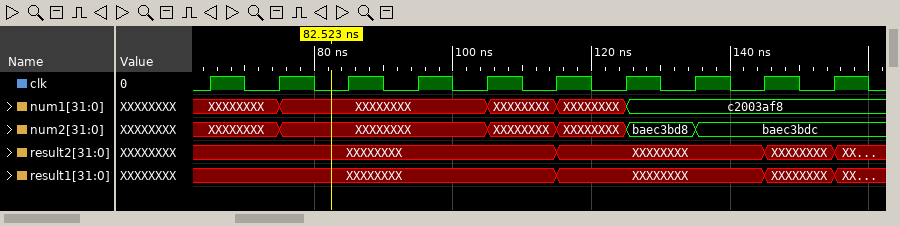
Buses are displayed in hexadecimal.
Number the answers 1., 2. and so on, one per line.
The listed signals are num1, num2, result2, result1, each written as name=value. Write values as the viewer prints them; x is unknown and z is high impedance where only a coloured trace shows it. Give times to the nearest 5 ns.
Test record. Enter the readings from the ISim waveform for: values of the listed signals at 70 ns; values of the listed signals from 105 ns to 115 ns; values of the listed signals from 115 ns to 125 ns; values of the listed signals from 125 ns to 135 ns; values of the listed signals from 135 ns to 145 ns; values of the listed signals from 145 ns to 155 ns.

1. num1=XXXXXXXX, num2=XXXXXXXX, result2=XXXXXXXX, result1=XXXXXXXX
2. num1=XXXXXXXX, num2=XXXXXXXX, result2=XXXXXXXX, result1=XXXXXXXX
3. num1=XXXXXXXX, num2=XXXXXXXX, result2=XXXXXXXX, result1=XXXXXXXX
4. num1=c2003af8, num2=baec3bd8, result2=XXXXXXXX, result1=XXXXXXXX
5. num1=c2003af8, num2=baec3bdc, result2=XXXXXXXX, result1=XXXXXXXX
6. num1=c2003af8, num2=baec3bdc, result2=XXXXXXXX, result1=XXXXXXXX
